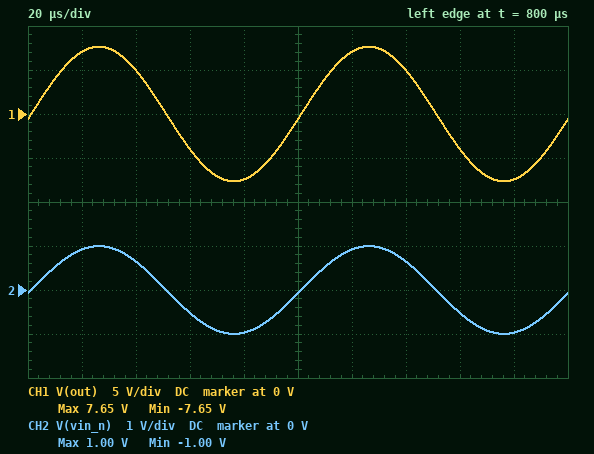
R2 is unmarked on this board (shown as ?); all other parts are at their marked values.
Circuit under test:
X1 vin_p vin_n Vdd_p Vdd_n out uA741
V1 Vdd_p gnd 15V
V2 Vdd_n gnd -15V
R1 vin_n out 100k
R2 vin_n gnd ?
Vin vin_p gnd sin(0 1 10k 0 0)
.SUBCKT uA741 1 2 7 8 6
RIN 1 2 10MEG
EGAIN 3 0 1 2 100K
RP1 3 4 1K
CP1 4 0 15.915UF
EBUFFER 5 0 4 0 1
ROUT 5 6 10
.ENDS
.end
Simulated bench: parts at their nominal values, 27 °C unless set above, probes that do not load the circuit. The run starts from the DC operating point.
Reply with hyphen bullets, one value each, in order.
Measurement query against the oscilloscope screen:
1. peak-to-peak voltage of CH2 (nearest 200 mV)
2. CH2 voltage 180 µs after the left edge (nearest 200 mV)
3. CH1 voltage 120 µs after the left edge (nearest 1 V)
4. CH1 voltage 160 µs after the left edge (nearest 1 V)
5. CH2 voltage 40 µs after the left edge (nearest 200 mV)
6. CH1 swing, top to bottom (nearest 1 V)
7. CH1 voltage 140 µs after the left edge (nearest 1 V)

- 2.0 V
- -1.0 V
- 7 V
- -4 V
- 600 mV
- 15 V
- 5 V
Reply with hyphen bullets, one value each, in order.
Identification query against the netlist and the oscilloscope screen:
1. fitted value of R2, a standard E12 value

- 15 kΩ
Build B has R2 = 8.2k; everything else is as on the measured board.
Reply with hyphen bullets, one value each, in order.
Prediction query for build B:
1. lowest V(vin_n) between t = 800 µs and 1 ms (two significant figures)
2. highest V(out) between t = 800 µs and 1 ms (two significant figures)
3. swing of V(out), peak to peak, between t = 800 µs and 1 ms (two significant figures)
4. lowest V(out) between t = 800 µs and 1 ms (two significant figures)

- -990 mV
- 13 V
- 26 V
- -13 V
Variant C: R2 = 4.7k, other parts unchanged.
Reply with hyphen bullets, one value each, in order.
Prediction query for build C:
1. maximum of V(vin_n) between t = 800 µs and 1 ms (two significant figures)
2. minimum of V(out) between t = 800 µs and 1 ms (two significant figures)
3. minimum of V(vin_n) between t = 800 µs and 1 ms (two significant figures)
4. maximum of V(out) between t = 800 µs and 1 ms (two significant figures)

- 980 mV
- -22 V
- -980 mV
- 22 V
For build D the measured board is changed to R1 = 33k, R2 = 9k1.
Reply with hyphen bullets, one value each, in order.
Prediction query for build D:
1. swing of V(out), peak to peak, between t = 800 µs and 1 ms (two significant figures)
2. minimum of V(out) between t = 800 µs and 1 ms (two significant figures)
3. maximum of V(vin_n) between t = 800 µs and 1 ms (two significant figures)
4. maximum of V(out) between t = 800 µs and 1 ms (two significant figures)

- 9.2 V
- -4.6 V
- 1.0 V
- 4.6 V
